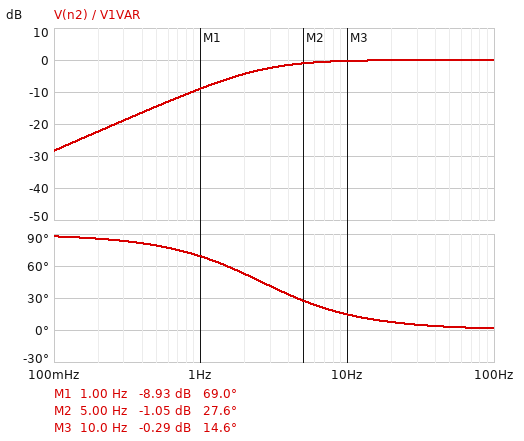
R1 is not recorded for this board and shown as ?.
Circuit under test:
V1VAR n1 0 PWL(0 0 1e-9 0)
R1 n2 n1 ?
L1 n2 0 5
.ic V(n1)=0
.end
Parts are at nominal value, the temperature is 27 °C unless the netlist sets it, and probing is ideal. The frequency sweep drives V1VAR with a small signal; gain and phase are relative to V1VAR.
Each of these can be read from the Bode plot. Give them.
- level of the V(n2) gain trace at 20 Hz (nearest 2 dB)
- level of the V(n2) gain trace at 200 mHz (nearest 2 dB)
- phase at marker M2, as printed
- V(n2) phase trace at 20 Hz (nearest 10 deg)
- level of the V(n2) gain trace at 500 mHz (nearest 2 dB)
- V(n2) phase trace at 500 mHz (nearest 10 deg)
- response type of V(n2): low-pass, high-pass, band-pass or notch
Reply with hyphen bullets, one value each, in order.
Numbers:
- 0 dB
- -22 dB
- 27.6 deg
- 10 deg
- -14 dB
- 80 deg
- high-pass
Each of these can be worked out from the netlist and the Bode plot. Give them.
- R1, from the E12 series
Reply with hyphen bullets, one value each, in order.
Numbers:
- 82 Ω
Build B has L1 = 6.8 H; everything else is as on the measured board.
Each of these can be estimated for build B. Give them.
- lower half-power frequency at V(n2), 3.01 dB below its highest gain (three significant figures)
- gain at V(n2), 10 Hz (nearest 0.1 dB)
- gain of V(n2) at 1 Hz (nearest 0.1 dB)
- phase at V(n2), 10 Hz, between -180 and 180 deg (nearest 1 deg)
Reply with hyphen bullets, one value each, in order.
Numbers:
- 1.92 Hz
- -0.2 dB
- -6.7 dB
- 11 deg
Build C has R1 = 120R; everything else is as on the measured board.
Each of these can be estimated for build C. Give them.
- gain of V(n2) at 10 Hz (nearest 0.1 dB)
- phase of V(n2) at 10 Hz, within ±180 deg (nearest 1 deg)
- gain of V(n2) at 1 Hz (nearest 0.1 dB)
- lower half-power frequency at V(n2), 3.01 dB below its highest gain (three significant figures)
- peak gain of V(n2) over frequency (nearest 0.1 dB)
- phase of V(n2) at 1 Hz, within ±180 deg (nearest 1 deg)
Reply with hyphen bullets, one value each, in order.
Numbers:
- -0.6 dB
- 21 deg
- -11.9 dB
- 3.82 Hz
- 0 dB
- 75 deg
